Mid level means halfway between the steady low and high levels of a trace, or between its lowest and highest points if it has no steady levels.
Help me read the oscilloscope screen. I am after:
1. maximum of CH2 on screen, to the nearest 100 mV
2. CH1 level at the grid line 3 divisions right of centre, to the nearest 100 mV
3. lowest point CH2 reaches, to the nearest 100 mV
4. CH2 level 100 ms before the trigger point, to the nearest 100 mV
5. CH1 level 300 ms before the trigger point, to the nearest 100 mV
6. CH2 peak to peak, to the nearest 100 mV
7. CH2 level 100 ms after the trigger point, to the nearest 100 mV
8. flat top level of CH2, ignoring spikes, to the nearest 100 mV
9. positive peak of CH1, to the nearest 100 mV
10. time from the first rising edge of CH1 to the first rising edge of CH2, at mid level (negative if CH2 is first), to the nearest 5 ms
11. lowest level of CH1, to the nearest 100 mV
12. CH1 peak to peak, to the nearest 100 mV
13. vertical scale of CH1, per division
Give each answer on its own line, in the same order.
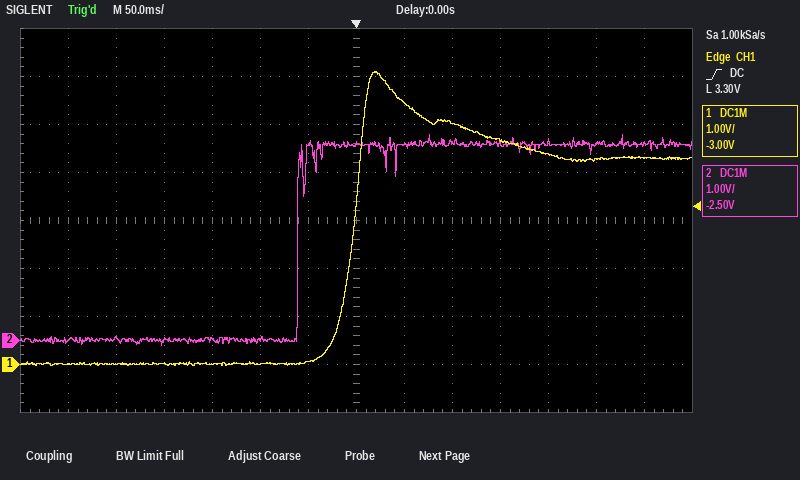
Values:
4.3 V
4.7 V
-100 mV
0.0 V
0.0 V
4.4 V
4.1 V
4.1 V
6.1 V
-60 ms
0.0 V
6.1 V
1 V
